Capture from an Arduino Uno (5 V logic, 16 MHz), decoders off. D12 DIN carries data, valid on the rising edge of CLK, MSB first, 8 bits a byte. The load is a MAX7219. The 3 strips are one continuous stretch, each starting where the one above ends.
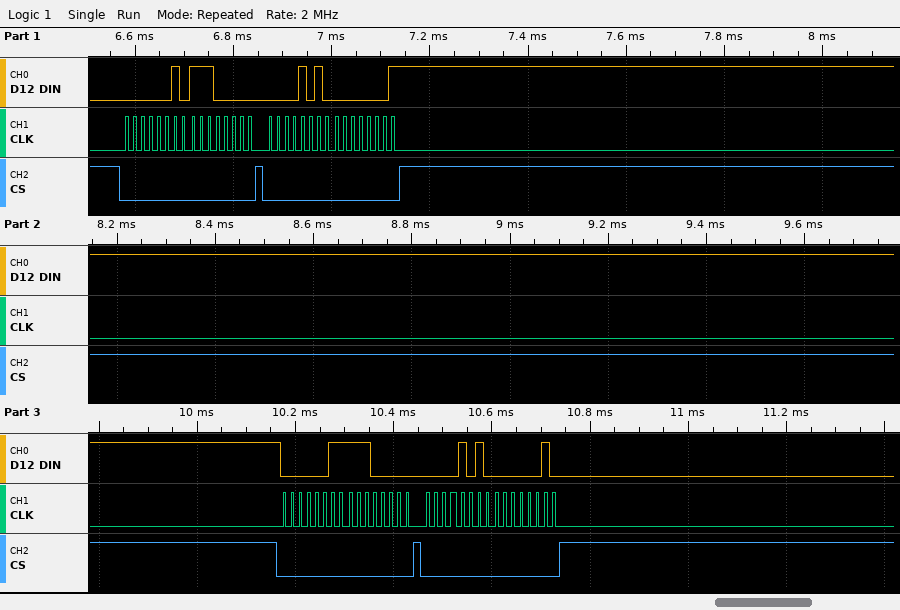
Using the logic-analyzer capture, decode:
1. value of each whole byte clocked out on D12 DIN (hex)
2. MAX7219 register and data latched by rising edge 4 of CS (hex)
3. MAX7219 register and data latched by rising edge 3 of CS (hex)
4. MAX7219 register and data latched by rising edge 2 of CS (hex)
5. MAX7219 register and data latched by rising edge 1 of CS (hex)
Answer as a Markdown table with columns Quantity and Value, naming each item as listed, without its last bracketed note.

| Quantity | Value |
|---|---|
| value of each whole byte clocked out on D12 DIN | 0x02 0xE0 0x0A 0x01 0x03 0xE0 0x0A 0x02 |
| MAX7219 register and data latched by rising edge 4 of CS | register 0xA, data 0x02 |
| MAX7219 register and data latched by rising edge 3 of CS | register 0x3, data 0xE0 |
| MAX7219 register and data latched by rising edge 2 of CS | register 0xA, data 0x01 |
| MAX7219 register and data latched by rising edge 1 of CS | register 0x2, data 0xE0 |
